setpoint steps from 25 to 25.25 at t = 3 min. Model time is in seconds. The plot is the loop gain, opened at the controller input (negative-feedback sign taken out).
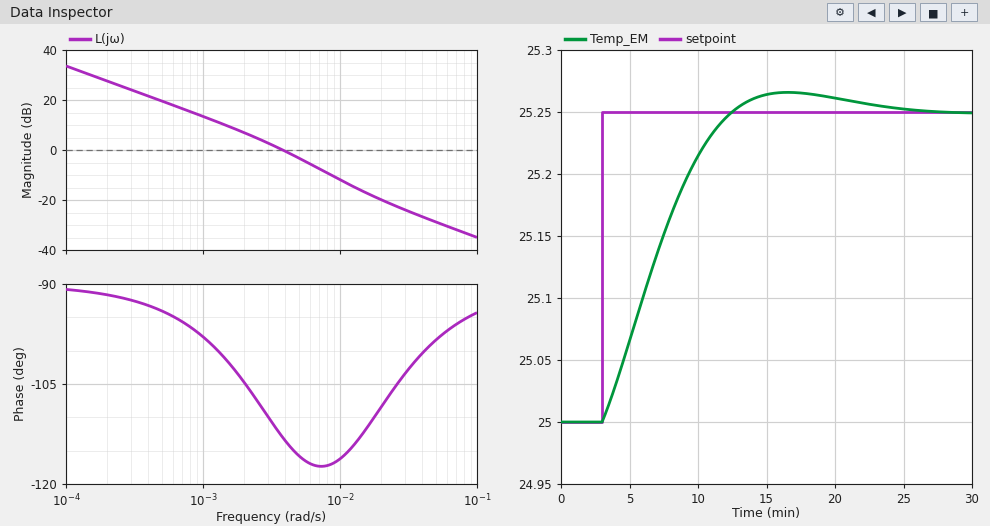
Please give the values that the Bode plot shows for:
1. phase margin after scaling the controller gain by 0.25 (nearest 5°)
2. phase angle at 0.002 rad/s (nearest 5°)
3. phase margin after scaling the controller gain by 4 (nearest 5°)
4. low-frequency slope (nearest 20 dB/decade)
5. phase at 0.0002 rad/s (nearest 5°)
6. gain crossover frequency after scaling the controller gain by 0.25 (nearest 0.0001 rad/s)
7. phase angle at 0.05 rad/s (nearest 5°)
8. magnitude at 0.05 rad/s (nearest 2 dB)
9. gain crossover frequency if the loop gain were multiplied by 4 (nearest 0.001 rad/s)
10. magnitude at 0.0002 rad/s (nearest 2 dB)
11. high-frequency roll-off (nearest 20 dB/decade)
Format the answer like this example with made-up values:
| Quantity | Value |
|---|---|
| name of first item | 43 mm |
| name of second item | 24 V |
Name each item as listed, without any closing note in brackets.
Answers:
| Quantity | Value |
|---|---|
| phase margin after scaling the controller gain by 0.25 | 80° |
| phase angle at 0.002 rad/s | -105° |
| phase margin after scaling the controller gain by 4 | 65° |
| low-frequency slope | -20 dB/decade |
| phase at 0.0002 rad/s | -90° |
| gain crossover frequency after scaling the controller gain by 0.25 | 0.0012 rad/s |
| phase angle at 0.05 rad/s | -100° |
| magnitude at 0.05 rad/s | -28 dB |
| gain crossover frequency if the loop gain were multiplied by 4 | 0.010 rad/s |
| magnitude at 0.0002 rad/s | 28 dB |
| high-frequency roll-off | -20 dB/decade |
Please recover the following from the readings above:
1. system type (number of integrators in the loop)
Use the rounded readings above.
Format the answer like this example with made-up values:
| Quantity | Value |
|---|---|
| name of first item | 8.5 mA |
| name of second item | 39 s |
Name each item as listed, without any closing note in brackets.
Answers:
| Quantity | Value |
|---|---|
| system type | 1 |
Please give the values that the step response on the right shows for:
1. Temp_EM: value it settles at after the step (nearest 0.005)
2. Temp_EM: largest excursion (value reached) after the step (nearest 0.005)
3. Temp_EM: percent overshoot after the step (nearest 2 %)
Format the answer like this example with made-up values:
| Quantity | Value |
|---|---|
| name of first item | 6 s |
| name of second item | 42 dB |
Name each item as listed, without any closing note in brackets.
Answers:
| Quantity | Value |
|---|---|
| Temp_EM: value it settles at after the step | 25.250 |
| Temp_EM: largest excursion (value reached) after the step | 25.265 |
| Temp_EM: percent overshoot after the step | 6 % |
